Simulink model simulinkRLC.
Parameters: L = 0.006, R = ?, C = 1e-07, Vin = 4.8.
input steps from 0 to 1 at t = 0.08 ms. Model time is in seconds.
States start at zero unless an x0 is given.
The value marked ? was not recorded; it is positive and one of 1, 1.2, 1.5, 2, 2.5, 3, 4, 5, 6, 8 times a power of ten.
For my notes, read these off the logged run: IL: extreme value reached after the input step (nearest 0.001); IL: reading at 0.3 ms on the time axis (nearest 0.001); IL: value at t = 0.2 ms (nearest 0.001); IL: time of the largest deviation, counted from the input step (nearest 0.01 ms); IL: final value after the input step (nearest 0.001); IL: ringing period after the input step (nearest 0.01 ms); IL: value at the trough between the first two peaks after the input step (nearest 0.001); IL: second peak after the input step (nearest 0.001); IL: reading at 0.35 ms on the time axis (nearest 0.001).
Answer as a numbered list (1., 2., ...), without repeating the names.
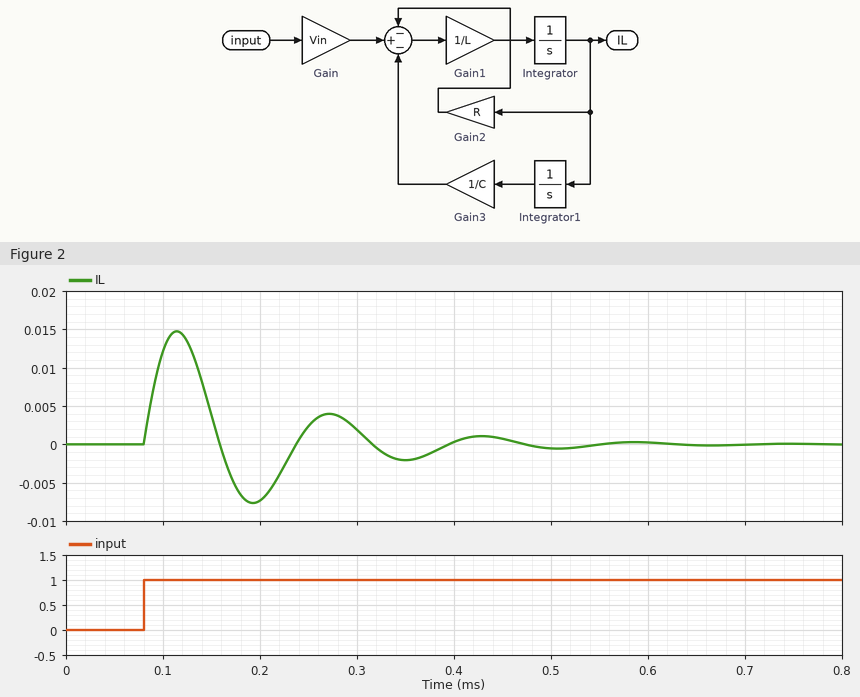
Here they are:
1. 0.015
2. 0.002
3. -0.007
4. 0.03 ms
5. 0.000
6. 0.16 ms
7. -0.008
8. 0.004
9. -0.002
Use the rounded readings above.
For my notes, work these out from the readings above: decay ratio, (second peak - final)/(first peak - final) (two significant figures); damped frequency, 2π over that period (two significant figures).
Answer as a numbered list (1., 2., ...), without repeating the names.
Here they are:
1. 0.27
2. 39 rad/ms
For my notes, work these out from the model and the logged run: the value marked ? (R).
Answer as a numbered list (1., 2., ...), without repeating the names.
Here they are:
1. 100
